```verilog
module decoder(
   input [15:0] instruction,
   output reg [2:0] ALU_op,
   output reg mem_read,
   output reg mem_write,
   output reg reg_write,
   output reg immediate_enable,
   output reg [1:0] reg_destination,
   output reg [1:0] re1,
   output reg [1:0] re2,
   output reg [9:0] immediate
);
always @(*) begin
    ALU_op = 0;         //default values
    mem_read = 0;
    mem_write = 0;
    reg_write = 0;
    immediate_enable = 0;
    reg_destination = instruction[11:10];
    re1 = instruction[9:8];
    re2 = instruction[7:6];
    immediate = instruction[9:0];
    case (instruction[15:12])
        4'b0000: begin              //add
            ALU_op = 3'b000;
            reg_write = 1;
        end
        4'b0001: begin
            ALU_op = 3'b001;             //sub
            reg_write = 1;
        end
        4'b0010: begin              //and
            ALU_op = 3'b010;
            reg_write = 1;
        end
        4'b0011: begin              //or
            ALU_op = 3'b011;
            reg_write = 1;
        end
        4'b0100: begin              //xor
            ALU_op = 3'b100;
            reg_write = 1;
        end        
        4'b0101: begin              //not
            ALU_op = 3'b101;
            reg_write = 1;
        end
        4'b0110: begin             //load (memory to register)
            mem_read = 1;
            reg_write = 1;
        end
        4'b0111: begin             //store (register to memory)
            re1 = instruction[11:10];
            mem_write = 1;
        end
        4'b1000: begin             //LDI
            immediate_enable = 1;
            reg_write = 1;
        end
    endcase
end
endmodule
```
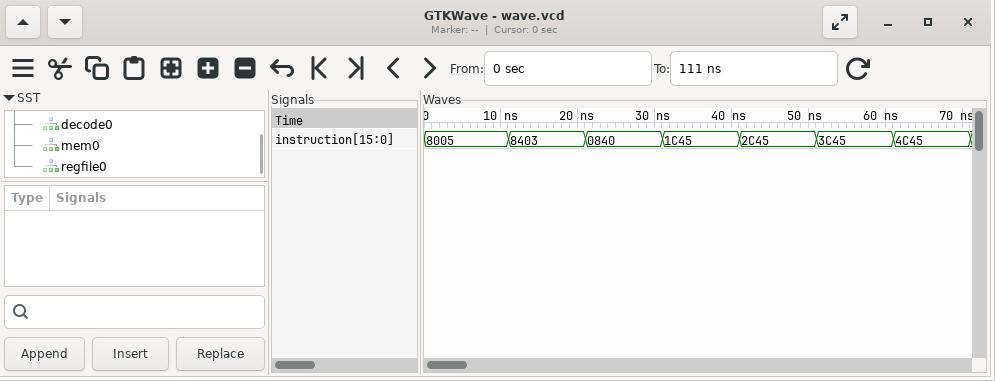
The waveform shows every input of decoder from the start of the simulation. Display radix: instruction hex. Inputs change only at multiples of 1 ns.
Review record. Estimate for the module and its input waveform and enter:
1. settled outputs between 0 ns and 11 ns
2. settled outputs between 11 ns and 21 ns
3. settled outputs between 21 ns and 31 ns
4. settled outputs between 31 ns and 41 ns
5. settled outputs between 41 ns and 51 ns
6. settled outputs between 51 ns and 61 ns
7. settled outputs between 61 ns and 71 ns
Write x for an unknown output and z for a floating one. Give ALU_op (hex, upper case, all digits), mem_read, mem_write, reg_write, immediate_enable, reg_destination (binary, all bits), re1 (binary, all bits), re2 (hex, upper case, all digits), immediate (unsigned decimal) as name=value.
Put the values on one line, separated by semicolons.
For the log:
ALU_op=0, mem_read=0, mem_write=0, reg_write=1, immediate_enable=1, reg_destination=00, re1=00, re2=0, immediate=5; ALU_op=0, mem_read=0, mem_write=0, reg_write=1, immediate_enable=1, reg_destination=01, re1=00, re2=0, immediate=3; ALU_op=0, mem_read=0, mem_write=0, reg_write=1, immediate_enable=0, reg_destination=10, re1=00, re2=1, immediate=64; ALU_op=1, mem_read=0, mem_write=0, reg_write=1, immediate_enable=0, reg_destination=11, re1=00, re2=1, immediate=69; ALU_op=2, mem_read=0, mem_write=0, reg_write=1, immediate_enable=0, reg_destination=11, re1=00, re2=1, immediate=69; ALU_op=3, mem_read=0, mem_write=0, reg_write=1, immediate_enable=0, reg_destination=11, re1=00, re2=1, immediate=69; ALU_op=4, mem_read=0, mem_write=0, reg_write=1, immediate_enable=0, reg_destination=11, re1=00, re2=1, immediate=69
